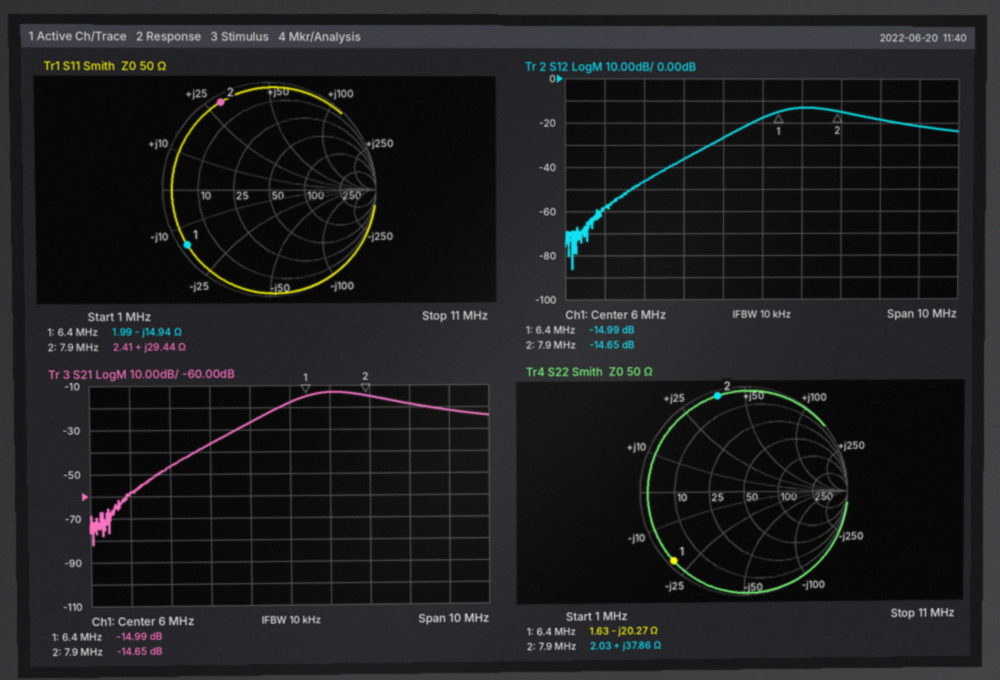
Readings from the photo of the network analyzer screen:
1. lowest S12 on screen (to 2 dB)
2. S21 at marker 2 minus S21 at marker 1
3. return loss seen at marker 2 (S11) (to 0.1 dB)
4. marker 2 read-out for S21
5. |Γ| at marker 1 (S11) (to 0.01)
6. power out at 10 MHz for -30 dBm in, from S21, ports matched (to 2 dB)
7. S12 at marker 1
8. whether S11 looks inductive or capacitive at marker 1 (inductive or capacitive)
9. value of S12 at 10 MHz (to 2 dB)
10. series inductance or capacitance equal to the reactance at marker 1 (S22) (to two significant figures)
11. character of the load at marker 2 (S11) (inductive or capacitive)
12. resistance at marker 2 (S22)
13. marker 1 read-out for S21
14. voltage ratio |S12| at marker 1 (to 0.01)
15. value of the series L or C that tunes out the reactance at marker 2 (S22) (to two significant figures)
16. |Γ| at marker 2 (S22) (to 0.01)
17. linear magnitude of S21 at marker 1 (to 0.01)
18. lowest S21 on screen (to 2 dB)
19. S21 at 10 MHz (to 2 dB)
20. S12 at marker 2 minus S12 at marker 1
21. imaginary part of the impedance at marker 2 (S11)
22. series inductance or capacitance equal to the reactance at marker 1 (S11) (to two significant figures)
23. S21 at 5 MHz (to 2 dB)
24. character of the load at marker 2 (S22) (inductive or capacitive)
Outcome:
-86 dB
0.34 dB
0.6 dB
-14.65 dB
0.93
-52 dBm
-14.99 dB
capacitive
-22 dB
1.2 nF
inductive
2.03 Ω
-14.99 dB
0.18
530 pF
0.95
0.18
-82 dB
-22 dB
0.34 dB
+29.44 Ω
1.7 nF
-26 dB
inductive
